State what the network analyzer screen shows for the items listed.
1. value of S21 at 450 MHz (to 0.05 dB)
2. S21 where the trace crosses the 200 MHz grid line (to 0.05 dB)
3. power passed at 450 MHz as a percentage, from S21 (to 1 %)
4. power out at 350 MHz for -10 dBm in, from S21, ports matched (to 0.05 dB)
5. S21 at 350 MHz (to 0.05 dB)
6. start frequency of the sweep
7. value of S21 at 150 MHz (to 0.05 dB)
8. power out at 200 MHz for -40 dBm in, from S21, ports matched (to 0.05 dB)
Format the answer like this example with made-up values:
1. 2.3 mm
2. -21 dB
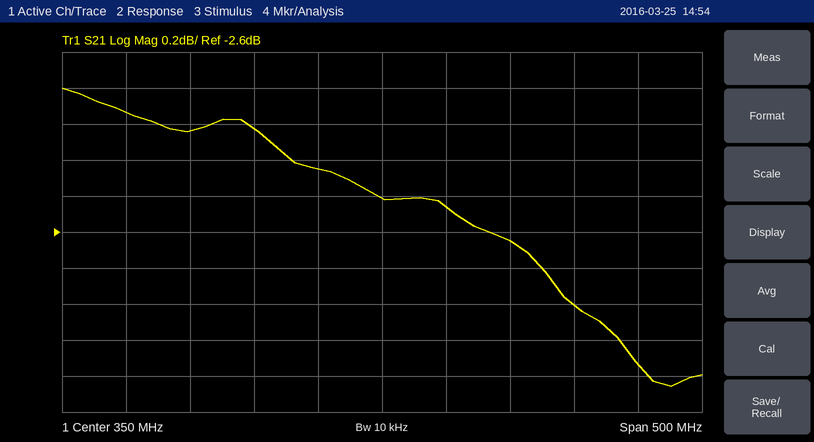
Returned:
1. -2.65 dB
2. -2.05 dB
3. 54 %
4. -12.40 dBm
5. -2.40 dB
6. 100 MHz
7. -1.95 dB
8. -42.05 dBm
